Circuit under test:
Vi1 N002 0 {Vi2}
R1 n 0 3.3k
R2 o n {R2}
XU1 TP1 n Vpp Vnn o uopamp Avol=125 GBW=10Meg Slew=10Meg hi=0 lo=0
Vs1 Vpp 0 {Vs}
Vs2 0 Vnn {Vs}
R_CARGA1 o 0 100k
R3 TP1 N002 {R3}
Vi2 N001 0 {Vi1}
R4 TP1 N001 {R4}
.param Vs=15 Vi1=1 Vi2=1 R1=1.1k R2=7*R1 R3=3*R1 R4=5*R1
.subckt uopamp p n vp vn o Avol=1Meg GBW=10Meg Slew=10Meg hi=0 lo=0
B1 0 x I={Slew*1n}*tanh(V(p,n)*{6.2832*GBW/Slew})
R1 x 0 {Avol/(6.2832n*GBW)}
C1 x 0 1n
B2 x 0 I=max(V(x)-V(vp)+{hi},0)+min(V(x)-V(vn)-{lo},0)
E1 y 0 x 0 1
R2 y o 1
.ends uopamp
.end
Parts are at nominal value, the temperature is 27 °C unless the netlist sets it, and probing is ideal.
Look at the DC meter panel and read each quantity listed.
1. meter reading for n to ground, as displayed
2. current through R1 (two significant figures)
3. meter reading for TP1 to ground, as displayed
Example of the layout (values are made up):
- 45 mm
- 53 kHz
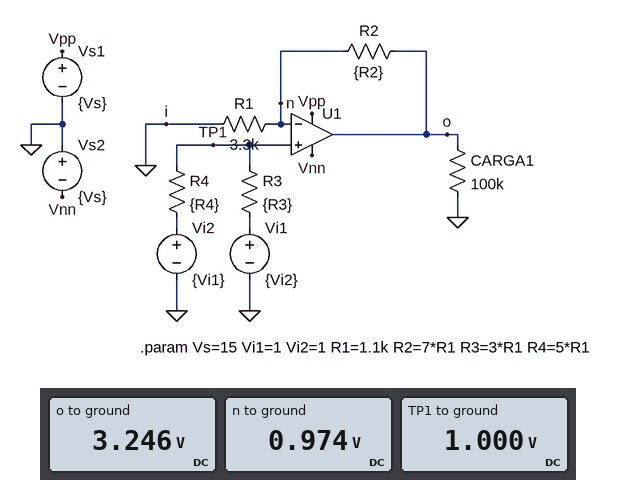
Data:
- 0.974 V
- 300 µA
- 1.000 V
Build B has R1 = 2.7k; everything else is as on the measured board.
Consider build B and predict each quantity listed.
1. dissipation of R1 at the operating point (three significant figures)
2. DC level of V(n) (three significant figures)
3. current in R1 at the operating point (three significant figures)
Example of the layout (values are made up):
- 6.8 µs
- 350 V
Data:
- 348 µW
- 970 mV
- 359 µA
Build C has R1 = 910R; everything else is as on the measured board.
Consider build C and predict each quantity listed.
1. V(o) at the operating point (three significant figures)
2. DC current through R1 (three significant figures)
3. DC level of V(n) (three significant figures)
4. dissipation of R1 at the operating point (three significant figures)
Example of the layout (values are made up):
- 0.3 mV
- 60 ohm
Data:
- 8.75 V
- 1.02 mA
- 925 mV
- 940 µW
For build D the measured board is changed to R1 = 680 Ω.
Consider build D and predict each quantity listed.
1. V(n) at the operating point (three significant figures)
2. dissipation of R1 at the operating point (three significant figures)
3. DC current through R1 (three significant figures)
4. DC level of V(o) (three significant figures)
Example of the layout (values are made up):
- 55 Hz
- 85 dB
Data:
- 900 mV
- 1.19 mW
- 1.32 mA
- 11.1 V
